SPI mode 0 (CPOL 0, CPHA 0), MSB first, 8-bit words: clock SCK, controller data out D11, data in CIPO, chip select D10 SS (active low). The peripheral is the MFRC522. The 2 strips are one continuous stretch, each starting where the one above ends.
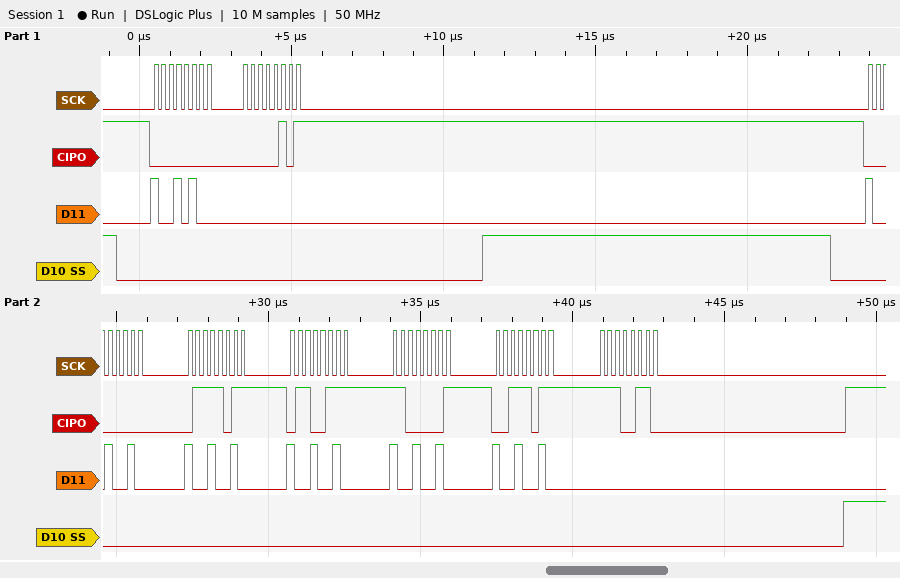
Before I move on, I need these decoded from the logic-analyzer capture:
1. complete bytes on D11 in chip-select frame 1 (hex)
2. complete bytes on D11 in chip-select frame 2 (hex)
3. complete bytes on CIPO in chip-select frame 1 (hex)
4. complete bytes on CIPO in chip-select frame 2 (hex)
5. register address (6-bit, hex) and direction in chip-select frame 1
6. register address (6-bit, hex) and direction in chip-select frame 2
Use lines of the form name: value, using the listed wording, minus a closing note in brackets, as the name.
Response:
complete bytes on D11 in chip-select frame 1: 94 00
complete bytes on D11 in chip-select frame 2: 92 92 92 92 92 00
complete bytes on CIPO in chip-select frame 1: 00 05
complete bytes on CIPO in chip-select frame 2: 00 7B 67 C1 3B E6
register address (6-bit, hex) and direction in chip-select frame 1: 0x0A read
register address (6-bit, hex) and direction in chip-select frame 2: 0x09 read
